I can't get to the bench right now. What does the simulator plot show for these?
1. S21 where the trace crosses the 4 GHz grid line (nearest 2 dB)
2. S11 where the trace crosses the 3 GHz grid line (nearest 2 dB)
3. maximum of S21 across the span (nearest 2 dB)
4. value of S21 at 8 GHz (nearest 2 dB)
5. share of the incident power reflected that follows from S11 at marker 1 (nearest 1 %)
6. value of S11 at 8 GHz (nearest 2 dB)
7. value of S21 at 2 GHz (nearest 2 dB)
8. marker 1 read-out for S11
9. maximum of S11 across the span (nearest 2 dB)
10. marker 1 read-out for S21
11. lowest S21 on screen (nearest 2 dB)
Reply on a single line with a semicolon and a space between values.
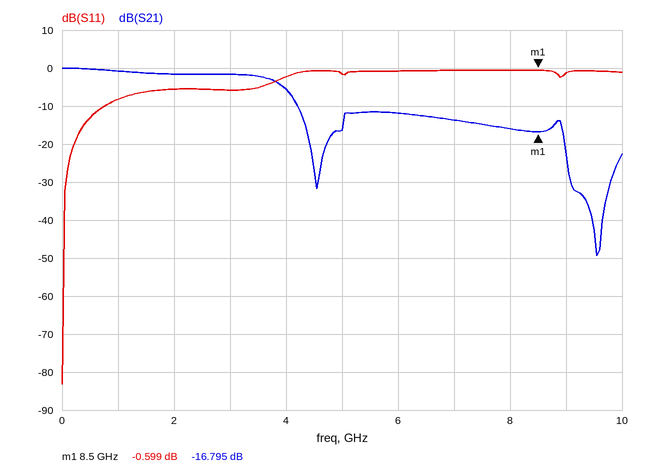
-6 dB; -6 dB; 0 dB; -16 dB; 87 %; 0 dB; -2 dB; -0.599 dB; 0 dB; -16.795 dB; -50 dB
